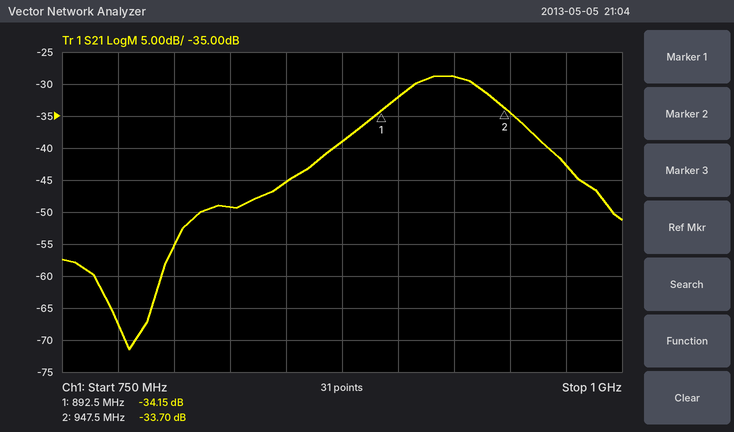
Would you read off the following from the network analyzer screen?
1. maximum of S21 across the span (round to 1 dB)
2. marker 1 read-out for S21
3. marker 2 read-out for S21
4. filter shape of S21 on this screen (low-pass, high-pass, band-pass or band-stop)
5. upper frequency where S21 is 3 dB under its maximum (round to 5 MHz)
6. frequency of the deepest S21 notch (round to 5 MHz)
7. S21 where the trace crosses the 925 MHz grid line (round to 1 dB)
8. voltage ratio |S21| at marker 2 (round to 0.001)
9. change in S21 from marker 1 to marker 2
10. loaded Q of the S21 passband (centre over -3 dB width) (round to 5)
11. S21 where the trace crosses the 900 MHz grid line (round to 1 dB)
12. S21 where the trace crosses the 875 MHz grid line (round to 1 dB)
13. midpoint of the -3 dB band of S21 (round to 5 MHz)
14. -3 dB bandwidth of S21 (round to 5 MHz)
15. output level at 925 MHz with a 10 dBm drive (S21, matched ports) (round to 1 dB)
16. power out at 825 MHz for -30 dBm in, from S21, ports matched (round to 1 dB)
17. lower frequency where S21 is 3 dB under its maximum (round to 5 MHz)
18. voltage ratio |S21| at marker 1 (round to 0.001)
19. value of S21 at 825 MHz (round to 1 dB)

-29 dB
-34.15 dB
-33.70 dB
band-pass
940 MHz
780 MHz
-29 dB
0.021
0.45 dB
25
-32 dB
-39 dB
920 MHz
40 MHz
-19 dBm
-79 dBm
900 MHz
0.020
-49 dB
